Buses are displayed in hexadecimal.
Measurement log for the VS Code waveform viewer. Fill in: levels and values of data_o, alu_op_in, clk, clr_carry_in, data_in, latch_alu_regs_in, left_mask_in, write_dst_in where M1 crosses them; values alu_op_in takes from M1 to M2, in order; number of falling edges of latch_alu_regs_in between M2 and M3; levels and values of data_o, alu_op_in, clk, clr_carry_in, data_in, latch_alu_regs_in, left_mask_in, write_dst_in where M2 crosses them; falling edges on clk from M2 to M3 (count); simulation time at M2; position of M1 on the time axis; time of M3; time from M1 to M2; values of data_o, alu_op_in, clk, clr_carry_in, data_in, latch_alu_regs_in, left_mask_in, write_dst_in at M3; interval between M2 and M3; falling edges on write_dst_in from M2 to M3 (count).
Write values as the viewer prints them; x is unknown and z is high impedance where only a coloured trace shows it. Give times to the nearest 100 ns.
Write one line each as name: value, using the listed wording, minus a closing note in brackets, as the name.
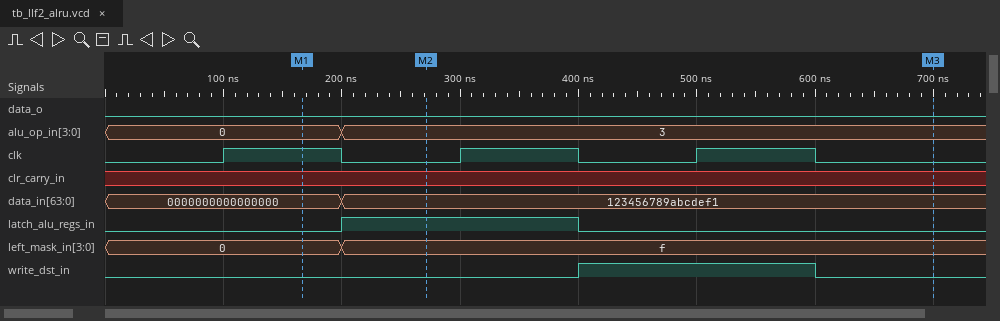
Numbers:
levels and values of data_o, alu_op_in, clk, clr_carry_in, data_in, latch_alu_regs_in, left_mask_in, write_dst_in where M1 crosses them: data_o=0, alu_op_in=0, clk=1, clr_carry_in=x, data_in=0000000000000000, latch_alu_regs_in=0, left_mask_in=0, write_dst_in=0
values alu_op_in takes from M1 to M2, in order: 0, 3
number of falling edges of latch_alu_regs_in between M2 and M3: 1
levels and values of data_o, alu_op_in, clk, clr_carry_in, data_in, latch_alu_regs_in, left_mask_in, write_dst_in where M2 crosses them: data_o=0, alu_op_in=3, clk=0, clr_carry_in=x, data_in=123456789abcdef1, latch_alu_regs_in=1, left_mask_in=f, write_dst_in=0
falling edges on clk from M2 to M3: 2
simulation time at M2: 300 ns
position of M1 on the time axis: 200 ns
time of M3: 700 ns
time from M1 to M2: 100 ns
values of data_o, alu_op_in, clk, clr_carry_in, data_in, latch_alu_regs_in, left_mask_in, write_dst_in at M3: data_o=0, alu_op_in=3, clk=0, clr_carry_in=x, data_in=123456789abcdef1, latch_alu_regs_in=0, left_mask_in=f, write_dst_in=0
interval between M2 and M3: 400 ns
falling edges on write_dst_in from M2 to M3: 1
